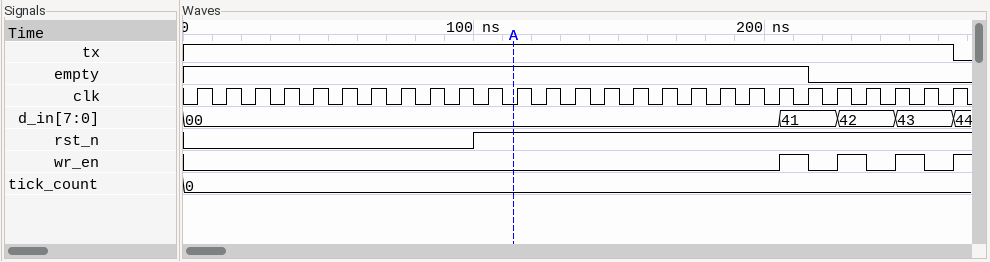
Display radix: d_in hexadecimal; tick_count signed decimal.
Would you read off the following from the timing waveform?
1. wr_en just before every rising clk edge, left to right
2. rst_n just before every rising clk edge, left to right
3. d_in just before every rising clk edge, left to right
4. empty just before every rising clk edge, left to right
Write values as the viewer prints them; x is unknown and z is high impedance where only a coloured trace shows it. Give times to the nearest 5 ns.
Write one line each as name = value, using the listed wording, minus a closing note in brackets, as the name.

wr_en just before every rising clk edge, left to right = 0 0 0 0 0 0 0 0 0 0 0 0 0 0 0 0 0 0 0 0 0 1 0 1 0 1 0
rst_n just before every rising clk edge, left to right = 0 0 0 0 0 0 0 0 0 0 1 1 1 1 1 1 1 1 1 1 1 1 1 1 1 1 1
d_in just before every rising clk edge, left to right = 00, 00, 00, 00, 00, 00, 00, 00, 00, 00, 00, 00, 00, 00, 00, 00, 00, 00, 00, 00, 00, 41, 41, 42, 42, 43, 43
empty just before every rising clk edge, left to right = 1 1 1 1 1 1 1 1 1 1 1 1 1 1 1 1 1 1 1 1 1 1 0 0 0 0 0
